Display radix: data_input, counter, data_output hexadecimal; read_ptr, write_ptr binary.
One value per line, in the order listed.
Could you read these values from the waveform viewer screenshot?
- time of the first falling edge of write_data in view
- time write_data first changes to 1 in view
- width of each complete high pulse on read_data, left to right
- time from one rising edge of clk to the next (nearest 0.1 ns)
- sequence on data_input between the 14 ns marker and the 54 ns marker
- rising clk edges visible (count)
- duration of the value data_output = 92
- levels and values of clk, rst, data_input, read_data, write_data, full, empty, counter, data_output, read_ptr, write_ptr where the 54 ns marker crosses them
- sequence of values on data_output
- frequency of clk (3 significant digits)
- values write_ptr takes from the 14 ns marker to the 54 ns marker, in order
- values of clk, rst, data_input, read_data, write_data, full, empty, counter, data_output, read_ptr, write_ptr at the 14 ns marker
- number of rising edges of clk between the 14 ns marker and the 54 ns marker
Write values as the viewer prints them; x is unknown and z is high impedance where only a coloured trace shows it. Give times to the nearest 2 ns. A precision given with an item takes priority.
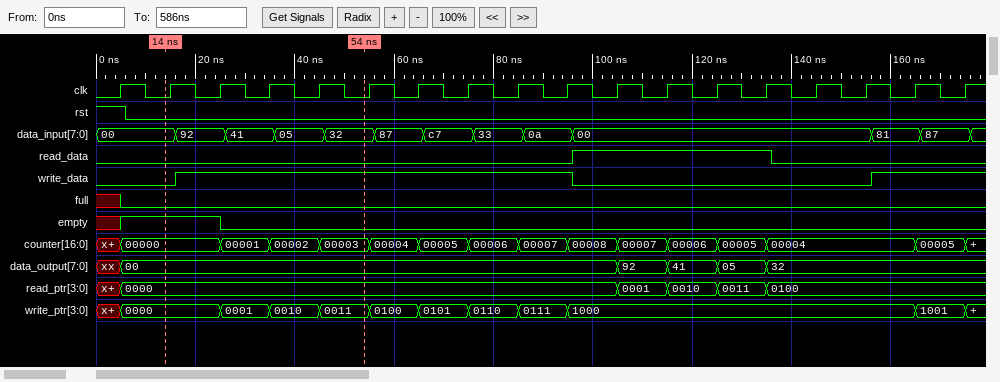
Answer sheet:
96 ns
16 ns
40 ns
10 ns
00, 92, 41, 05, 32
18
10 ns
clk=0, rst=0, data_input=32, read_data=0, write_data=1, full=0, empty=0, counter=00003, data_output=00, read_ptr=0000, write_ptr=0011
xx, 00, 92, 41, 05, 32
100 MHz
0000, 0001, 0010, 0011
clk=0, rst=0, data_input=00, read_data=0, write_data=0, full=0, empty=1, counter=00000, data_output=00, read_ptr=0000, write_ptr=0000
4
